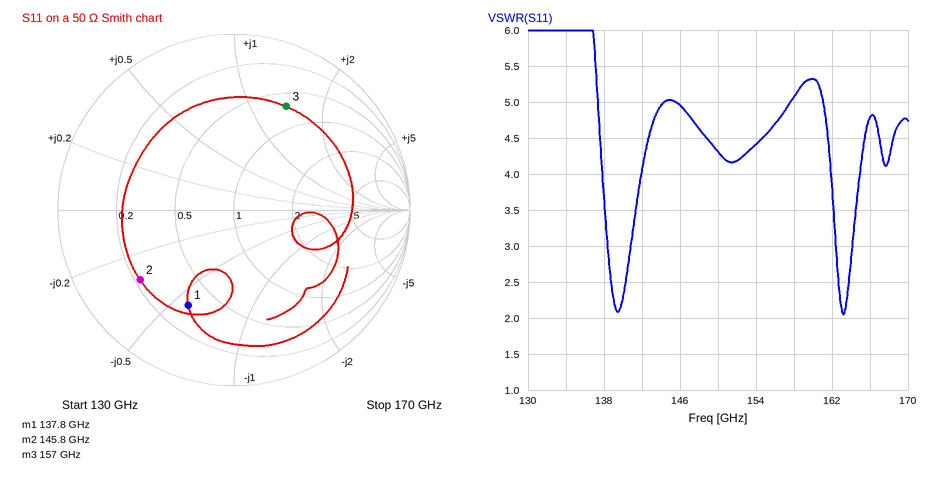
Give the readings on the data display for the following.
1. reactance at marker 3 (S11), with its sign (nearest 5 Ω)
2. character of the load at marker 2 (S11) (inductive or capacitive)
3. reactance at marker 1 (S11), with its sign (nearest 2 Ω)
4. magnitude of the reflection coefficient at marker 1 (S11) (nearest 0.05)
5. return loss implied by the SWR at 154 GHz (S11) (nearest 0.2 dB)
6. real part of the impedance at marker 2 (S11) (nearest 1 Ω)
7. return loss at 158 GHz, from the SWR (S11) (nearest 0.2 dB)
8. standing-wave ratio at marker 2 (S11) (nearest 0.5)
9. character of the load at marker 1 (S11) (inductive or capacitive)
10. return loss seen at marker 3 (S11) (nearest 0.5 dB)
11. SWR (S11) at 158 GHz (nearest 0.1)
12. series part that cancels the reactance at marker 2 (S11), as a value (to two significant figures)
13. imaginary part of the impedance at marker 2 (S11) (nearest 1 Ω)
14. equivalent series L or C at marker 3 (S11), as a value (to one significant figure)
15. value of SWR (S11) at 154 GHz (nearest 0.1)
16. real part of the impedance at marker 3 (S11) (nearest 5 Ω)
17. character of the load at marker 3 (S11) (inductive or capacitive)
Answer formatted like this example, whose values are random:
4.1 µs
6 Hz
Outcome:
+70 Ω
capacitive
-28 Ω
0.60
4.0 dB
11 Ω
3.4 dB
5.0
capacitive
3.5 dB
5.1
17 pH
-16 Ω
70 pH
4.4
35 Ω
inductive
